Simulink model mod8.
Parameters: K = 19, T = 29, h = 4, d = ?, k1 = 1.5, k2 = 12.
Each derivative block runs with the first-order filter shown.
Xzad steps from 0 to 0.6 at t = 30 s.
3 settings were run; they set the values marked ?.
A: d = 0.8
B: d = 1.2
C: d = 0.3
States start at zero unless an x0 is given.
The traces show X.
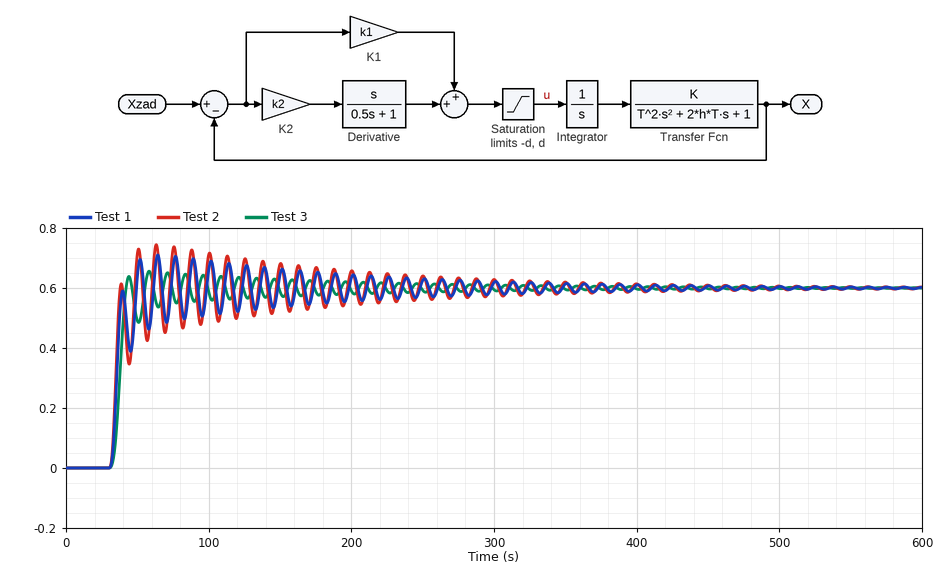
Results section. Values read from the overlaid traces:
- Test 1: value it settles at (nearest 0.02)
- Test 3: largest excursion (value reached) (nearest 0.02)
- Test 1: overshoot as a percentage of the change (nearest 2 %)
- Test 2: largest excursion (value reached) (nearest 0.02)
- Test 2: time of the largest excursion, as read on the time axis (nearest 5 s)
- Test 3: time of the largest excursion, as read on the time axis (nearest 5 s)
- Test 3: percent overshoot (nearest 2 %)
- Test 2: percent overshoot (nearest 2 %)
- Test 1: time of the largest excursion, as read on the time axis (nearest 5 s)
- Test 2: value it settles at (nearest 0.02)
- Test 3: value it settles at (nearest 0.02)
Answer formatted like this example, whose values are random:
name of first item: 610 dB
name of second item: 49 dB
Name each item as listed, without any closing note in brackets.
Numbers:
Test 1: value it settles at: 0.60
Test 3: largest excursion (value reached): 0.66
Test 1: overshoot as a percentage of the change: 18 %
Test 2: largest excursion (value reached): 0.74
Test 2: time of the largest excursion, as read on the time axis: 65 s
Test 3: time of the largest excursion, as read on the time axis: 60 s
Test 3: percent overshoot: 10 %
Test 2: percent overshoot: 24 %
Test 1: time of the largest excursion, as read on the time axis: 65 s
Test 2: value it settles at: 0.60
Test 3: value it settles at: 0.60
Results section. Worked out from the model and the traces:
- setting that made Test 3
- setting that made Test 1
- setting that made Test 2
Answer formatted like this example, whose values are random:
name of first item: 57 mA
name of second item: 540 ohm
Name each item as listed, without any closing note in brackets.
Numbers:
setting that made Test 3: C
setting that made Test 1: A
setting that made Test 2: B
